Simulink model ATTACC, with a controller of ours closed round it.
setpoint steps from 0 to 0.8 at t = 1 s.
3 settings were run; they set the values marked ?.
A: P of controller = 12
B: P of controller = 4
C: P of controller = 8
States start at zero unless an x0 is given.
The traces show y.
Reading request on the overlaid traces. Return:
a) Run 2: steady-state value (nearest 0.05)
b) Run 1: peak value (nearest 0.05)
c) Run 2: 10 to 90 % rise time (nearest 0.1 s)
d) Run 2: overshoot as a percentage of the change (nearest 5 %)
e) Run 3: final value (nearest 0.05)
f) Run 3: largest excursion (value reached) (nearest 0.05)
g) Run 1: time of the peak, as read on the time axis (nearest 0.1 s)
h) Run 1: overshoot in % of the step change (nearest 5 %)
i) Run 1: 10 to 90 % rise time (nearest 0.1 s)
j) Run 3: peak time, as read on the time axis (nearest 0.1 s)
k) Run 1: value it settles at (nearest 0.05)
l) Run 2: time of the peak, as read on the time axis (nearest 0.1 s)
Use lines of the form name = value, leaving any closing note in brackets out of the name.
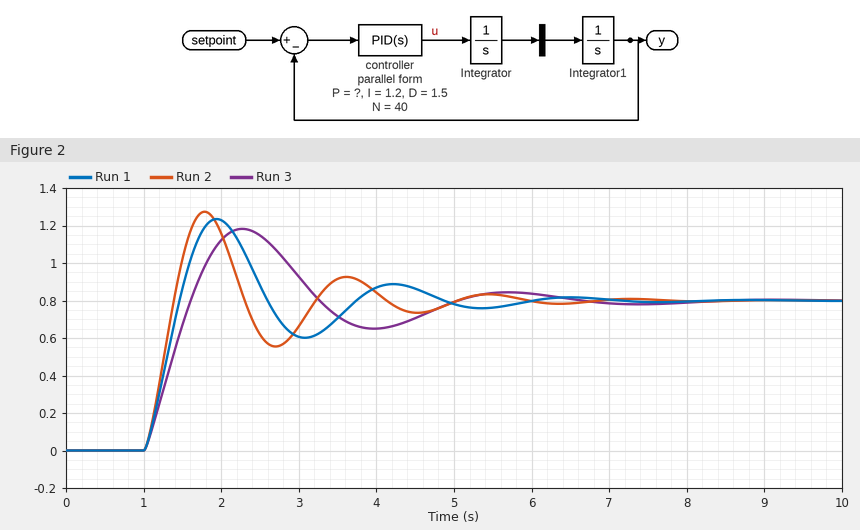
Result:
Run 2: steady-state value = 0.80
Run 1: peak value = 1.25
Run 2: 10 to 90 % rise time = 0.3 s
Run 2: overshoot as a percentage of the change = 60 %
Run 3: final value = 0.80
Run 3: largest excursion (value reached) = 1.20
Run 1: time of the peak, as read on the time axis = 1.9 s
Run 1: overshoot in % of the step change = 55 %
Run 1: 10 to 90 % rise time = 0.3 s
Run 3: peak time, as read on the time axis = 2.3 s
Run 1: value it settles at = 0.80
Run 2: time of the peak, as read on the time axis = 1.8 s
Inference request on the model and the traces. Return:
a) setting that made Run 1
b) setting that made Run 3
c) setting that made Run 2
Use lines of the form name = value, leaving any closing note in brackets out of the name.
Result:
setting that made Run 1 = C
setting that made Run 3 = B
setting that made Run 2 = A
